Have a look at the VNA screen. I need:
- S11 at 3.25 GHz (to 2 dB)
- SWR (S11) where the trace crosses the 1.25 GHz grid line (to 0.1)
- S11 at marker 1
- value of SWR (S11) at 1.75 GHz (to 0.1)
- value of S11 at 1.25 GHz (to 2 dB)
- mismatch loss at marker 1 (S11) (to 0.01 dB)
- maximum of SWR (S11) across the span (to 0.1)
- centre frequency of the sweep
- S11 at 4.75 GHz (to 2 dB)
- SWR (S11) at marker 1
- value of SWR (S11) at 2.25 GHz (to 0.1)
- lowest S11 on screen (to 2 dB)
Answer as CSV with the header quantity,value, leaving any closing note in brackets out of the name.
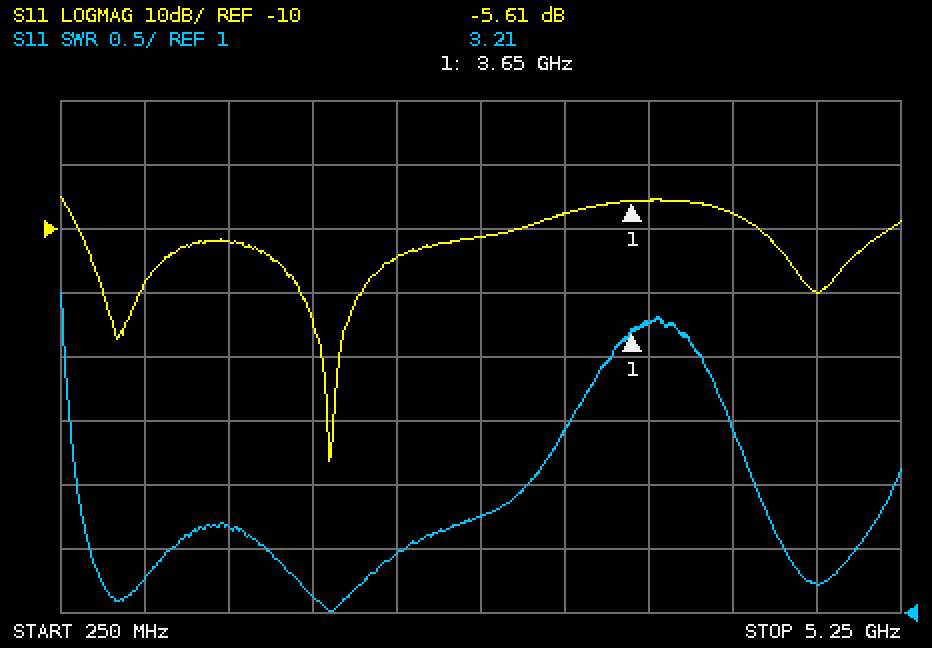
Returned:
quantity,value
S11 at 3.25 GHz,-8 dB
SWR (S11) where the trace crosses the 1.25 GHz grid line,1.7
S11 at marker 1,-5.61 dB
value of SWR (S11) at 1.75 GHz,1.1
value of S11 at 1.25 GHz,-12 dB
mismatch loss at marker 1 (S11),1.40 dB
maximum of SWR (S11) across the span,3.5
centre frequency of the sweep,2.75 GHz
S11 at 4.75 GHz,-20 dB
SWR (S11) at marker 1,3.21
value of SWR (S11) at 2.25 GHz,1.5
lowest S11 on screen,-46 dB
